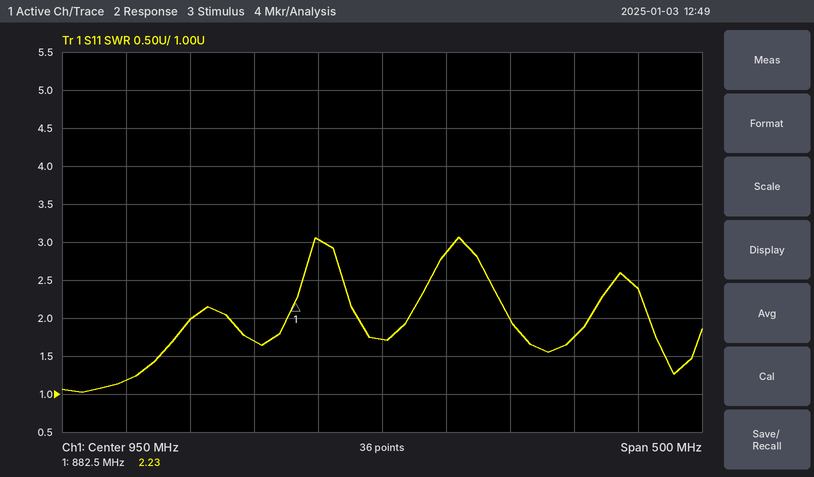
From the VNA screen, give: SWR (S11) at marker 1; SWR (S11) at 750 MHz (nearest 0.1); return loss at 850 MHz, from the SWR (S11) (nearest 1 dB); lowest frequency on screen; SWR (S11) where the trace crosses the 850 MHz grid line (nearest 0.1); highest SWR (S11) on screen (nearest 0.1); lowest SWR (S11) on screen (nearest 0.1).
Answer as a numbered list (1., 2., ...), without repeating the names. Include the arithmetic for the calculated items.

1. 2.23
2. 1.2
3. −20 log10((1.7 − 1)/(1.7 + 1)) ≈ 12 dB
4. 700 MHz
5. 1.7
6. 3.1
7. 1.0
